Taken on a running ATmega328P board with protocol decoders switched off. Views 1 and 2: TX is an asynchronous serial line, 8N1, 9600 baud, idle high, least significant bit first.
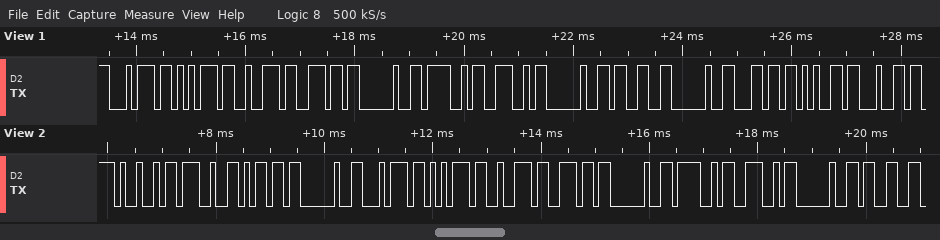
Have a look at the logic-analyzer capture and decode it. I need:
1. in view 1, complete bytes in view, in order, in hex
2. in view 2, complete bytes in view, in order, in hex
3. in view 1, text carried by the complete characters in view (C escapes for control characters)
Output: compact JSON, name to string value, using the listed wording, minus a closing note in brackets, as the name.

{"in view 1, complete bytes in view, in order, in hex": "74 75 72 6E 20 4F 4E 20 33 20 6C 65 64", "in view 2, complete bytes in view, in order, in hex": "49 27 6D 20 74 75 72 6E 20 4F 4E 20 33", "in view 1, text carried by the complete characters in view": "\"turn ON 3 led\""}
